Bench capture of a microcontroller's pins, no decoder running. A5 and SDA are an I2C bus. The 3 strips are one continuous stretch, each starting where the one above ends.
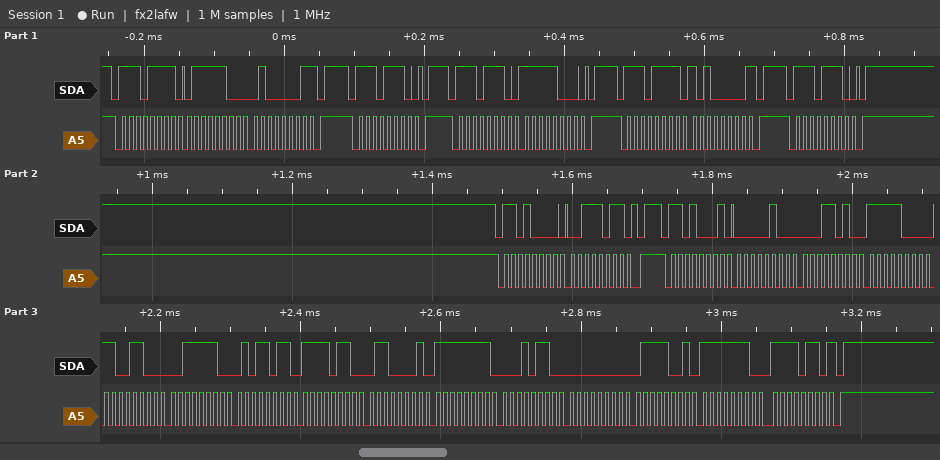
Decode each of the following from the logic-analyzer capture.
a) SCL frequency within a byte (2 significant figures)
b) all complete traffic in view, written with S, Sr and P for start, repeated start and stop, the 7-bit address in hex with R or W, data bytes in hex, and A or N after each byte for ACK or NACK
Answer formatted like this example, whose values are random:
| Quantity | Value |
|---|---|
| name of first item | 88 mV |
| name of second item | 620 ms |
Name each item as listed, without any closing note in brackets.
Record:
| Quantity | Value |
|---|---|
| SCL frequency within a byte | 100 kHz |
| all complete traffic in view, written with S, Sr and P for start, repeated start and stop, the 7-bit address in hex with R or W, data bytes in hex, and A or N after each byte for ACK or NACK | S 77R A 7C A 41 N P S 77W A P S 77W A F8 A P S 77R A A0 N P S 77W A P S 68W A 3B A P S 68R A 04 A 1A A F8 A CC A 3E A 5B A F6 A 61 A FF A 16 A 00 A 79 A FE A F6 N P |
